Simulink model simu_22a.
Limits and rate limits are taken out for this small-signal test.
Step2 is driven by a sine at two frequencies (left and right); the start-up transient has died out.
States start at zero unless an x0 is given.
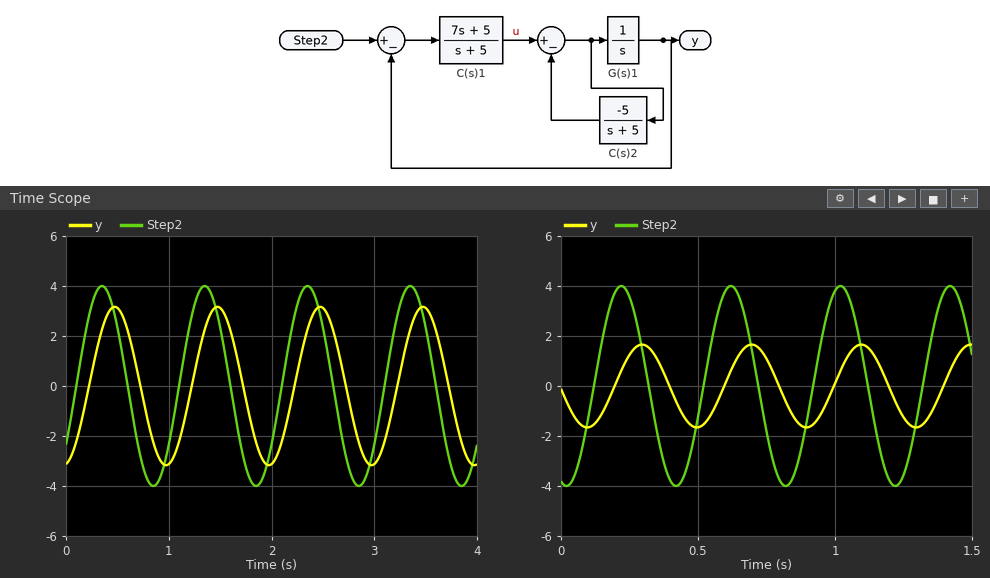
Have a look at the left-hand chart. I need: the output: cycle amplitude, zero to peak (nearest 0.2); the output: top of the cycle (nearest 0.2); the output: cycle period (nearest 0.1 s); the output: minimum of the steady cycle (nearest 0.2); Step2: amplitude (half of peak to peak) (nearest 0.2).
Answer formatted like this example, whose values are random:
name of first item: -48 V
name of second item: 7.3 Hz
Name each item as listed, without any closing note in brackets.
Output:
the output: cycle amplitude, zero to peak: 3.2
the output: top of the cycle: 3.2
the output: cycle period: 1.0 s
the output: minimum of the steady cycle: -3.2
Step2: amplitude (half of peak to peak): 4.0
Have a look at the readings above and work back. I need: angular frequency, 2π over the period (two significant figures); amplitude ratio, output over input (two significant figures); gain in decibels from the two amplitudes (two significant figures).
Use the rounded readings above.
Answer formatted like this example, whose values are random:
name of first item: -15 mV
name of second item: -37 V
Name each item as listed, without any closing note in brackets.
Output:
angular frequency, 2π over the period: 6.3 rad/s
amplitude ratio, output over input: 0.80
gain in decibels from the two amplitudes: -1.9 dB
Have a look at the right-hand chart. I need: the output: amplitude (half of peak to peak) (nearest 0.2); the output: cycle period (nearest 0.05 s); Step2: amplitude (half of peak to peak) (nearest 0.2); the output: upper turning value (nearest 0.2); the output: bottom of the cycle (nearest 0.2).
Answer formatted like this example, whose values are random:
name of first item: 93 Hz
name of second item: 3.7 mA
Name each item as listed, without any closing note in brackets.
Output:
the output: amplitude (half of peak to peak): 1.6
the output: cycle period: 0.40 s
Step2: amplitude (half of peak to peak): 4.0
the output: upper turning value: 1.6
the output: bottom of the cycle: -1.6
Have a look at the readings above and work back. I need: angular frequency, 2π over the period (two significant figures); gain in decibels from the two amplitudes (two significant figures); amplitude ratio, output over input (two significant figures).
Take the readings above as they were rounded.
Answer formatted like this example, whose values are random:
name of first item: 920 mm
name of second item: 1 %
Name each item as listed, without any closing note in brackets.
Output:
angular frequency, 2π over the period: 16 rad/s
gain in decibels from the two amplitudes: -8.0 dB
amplitude ratio, output over input: 0.40
